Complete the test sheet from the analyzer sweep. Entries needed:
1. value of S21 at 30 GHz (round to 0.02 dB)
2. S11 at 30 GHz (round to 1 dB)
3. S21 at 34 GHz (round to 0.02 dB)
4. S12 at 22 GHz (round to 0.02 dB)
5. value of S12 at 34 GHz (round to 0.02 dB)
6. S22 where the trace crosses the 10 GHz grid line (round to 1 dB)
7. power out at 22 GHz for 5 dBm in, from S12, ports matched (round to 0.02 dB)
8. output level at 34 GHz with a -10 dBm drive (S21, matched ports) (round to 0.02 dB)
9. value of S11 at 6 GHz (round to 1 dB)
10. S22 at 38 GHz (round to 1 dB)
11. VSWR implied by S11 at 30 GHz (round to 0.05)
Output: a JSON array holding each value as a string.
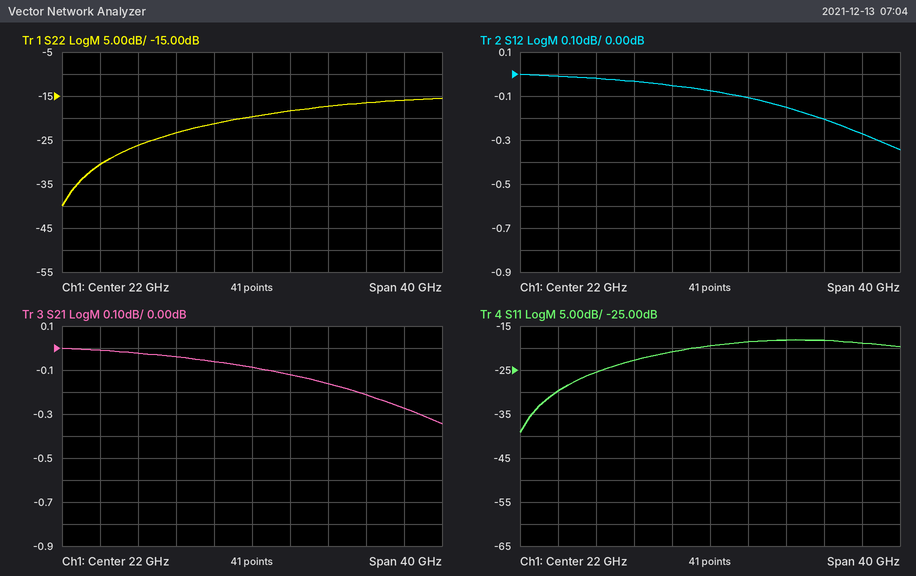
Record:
["-0.16 dB", "-18 dB", "-0.22 dB", "-0.08 dB", "-0.20 dB", "-26 dB", "4.92 dBm", "-10.22 dBm", "-30 dB", "-16 dB", "1.30"]
